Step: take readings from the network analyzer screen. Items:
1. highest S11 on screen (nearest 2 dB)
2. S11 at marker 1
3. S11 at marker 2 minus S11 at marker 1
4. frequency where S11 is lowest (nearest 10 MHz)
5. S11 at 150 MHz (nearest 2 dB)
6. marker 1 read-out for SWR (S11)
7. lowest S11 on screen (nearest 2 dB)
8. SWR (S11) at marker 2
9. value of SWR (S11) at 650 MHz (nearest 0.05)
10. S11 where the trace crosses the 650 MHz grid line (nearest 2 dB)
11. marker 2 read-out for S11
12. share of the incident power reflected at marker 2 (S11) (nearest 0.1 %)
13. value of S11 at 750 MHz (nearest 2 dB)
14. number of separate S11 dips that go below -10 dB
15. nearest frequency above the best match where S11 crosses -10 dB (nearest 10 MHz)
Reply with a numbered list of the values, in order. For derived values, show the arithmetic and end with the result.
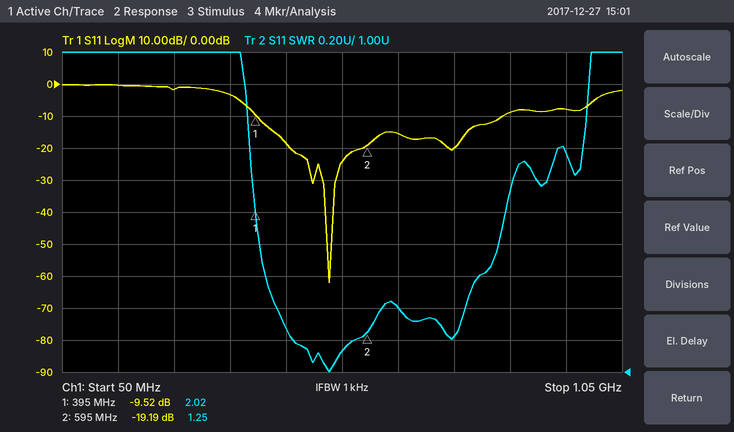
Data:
1. 0 dB
2. -9.52 dB
3. -19.19 − (-9.52) = -9.67 dB
4. 530 MHz
5. 0 dB
6. 2.02
7. -62 dB
8. 1.25
9. 1.40
10. -16 dB
11. -19.19 dB
12. 10^(-19.19/10) ≈ 1.2 %
13. -20 dB
14. 3
15. 840 MHz
